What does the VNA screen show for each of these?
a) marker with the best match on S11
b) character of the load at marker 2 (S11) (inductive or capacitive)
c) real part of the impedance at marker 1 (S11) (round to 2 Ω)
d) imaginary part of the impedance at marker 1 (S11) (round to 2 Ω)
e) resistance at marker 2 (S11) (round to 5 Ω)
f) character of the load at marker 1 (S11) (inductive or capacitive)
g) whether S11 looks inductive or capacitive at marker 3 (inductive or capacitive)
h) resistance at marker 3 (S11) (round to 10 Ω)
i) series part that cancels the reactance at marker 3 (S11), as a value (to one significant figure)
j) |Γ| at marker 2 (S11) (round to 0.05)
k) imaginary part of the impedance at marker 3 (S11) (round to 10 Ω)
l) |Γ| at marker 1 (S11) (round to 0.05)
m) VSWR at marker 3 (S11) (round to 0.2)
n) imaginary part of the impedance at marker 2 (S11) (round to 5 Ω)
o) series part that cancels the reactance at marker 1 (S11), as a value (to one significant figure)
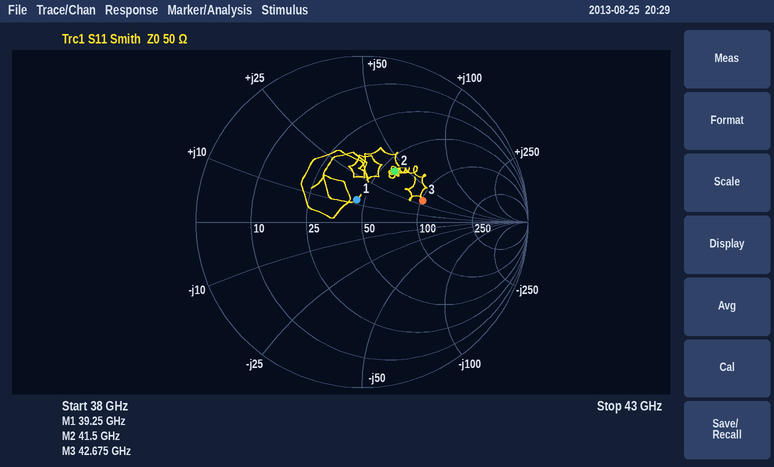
marker 1
inductive
46 Ω
+12 Ω
60 Ω
inductive
inductive
100 Ω
100 fF
0.35
+30 Ω
0.15
2.2
+40 Ω
300 fF
